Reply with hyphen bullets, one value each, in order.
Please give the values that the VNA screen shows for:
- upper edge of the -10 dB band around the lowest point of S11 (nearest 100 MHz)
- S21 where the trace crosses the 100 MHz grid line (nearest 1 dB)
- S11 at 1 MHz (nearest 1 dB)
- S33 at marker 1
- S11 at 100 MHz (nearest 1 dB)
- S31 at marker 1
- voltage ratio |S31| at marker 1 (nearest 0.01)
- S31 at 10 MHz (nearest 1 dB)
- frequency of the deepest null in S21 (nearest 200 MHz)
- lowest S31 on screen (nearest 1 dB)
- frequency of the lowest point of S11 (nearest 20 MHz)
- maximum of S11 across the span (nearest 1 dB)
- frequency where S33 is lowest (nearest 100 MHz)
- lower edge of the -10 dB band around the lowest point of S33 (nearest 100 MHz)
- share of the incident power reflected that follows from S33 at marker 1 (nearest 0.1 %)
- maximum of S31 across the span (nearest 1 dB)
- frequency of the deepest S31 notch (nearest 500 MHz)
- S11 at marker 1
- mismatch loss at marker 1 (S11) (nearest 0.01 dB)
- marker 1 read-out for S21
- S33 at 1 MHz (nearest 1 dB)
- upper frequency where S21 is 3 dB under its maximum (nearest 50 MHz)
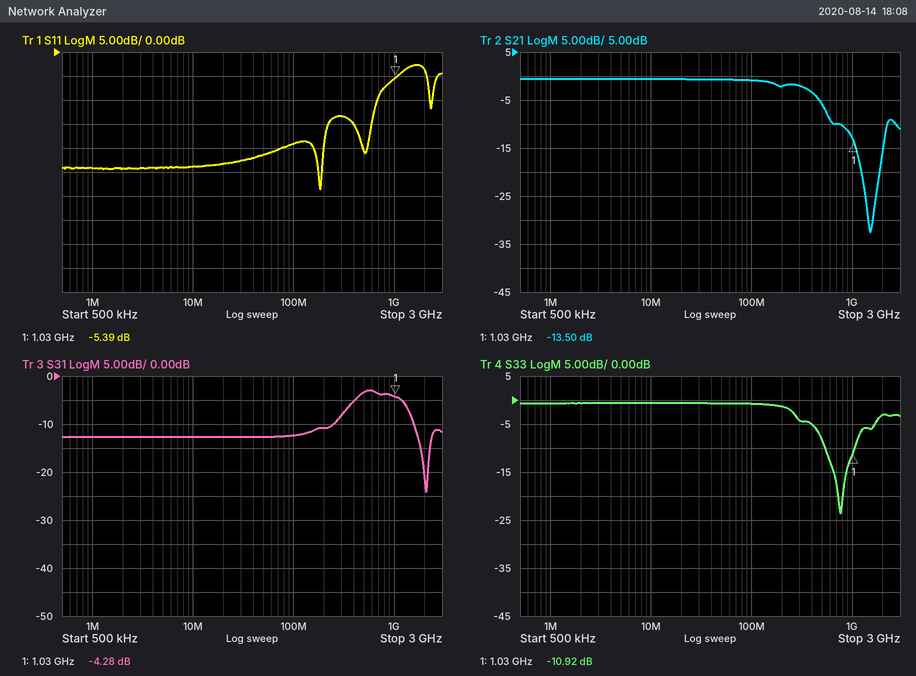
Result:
- 700 MHz
- -1 dB
- -24 dB
- -10.92 dB
- -19 dB
- -4.28 dB
- 0.61
- -13 dB
- 1.6 GHz
- -24 dB
- 180 MHz
- -3 dB
- 800 MHz
- 500 MHz
- 8.1 %
- -3 dB
- 2.0 GHz
- -5.39 dB
- 1.48 dB
- -13.50 dB
- -1 dB
- 400 MHz
